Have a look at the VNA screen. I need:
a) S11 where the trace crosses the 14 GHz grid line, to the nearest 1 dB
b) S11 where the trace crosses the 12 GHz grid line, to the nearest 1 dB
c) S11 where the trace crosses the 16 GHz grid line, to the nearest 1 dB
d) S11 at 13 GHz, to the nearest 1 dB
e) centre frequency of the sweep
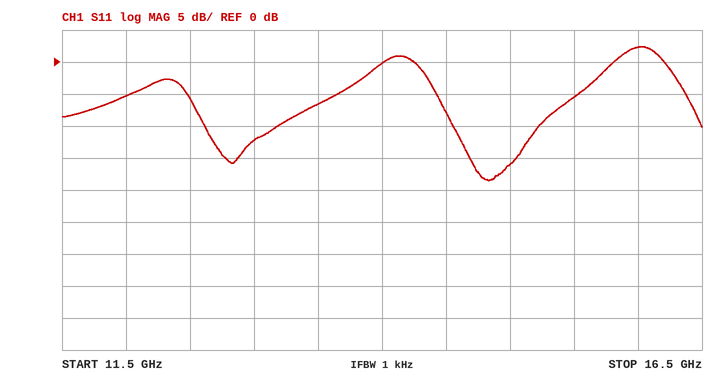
0 dB
-5 dB
2 dB
-12 dB
14 GHz
